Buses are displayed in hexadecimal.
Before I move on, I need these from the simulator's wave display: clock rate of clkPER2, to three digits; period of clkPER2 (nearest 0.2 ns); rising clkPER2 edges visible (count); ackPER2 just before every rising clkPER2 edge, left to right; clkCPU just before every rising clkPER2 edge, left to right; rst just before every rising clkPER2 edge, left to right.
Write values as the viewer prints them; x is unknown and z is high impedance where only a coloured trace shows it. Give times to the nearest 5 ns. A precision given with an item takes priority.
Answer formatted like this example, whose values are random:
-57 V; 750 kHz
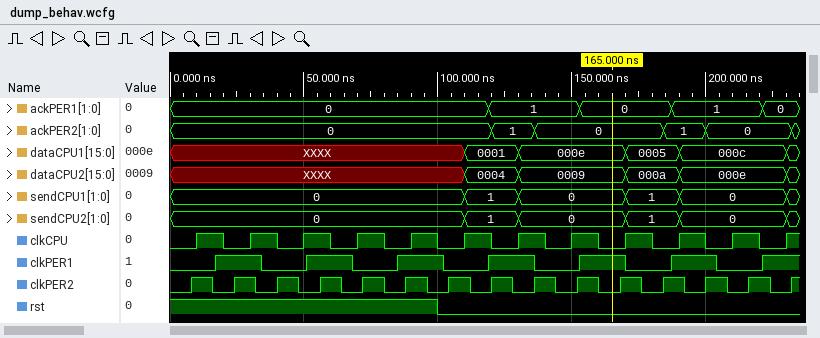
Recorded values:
62.5 MHz; 16 ns; 15; 0, 0, 0, 0, 0, 0, 0, 0, 1, 0, 0, 0, 1, 0, 0; 0 0 1 1 1 0 0 1 1 1 0 0 1 1 1; 1 1 1 1 1 1 0 0 0 0 0 0 0 0 0
